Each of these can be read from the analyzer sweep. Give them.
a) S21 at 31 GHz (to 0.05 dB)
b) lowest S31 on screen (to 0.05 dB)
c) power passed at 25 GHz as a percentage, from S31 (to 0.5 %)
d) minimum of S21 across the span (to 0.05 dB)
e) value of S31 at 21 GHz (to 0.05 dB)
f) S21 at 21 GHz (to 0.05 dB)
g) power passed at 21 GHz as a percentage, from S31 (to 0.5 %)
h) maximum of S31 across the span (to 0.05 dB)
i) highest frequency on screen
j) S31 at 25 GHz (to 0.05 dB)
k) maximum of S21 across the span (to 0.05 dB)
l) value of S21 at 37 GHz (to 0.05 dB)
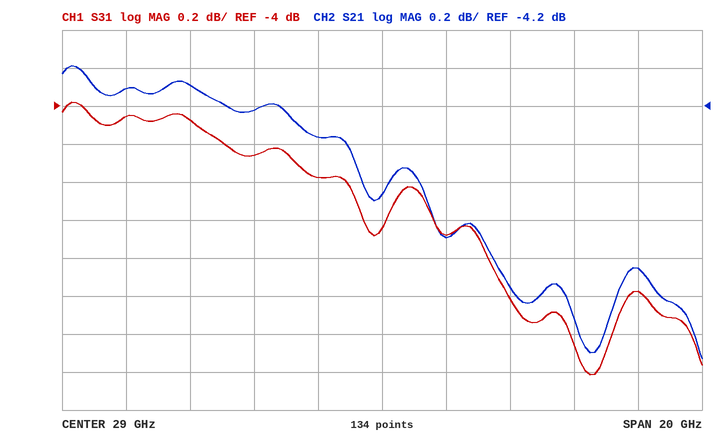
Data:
-4.90 dB
-5.40 dB
37.5 %
-5.55 dB
-4.05 dB
-4.10 dB
39.5 %
-4.00 dB
39 GHz
-4.25 dB
-4.00 dB
-5.05 dB
